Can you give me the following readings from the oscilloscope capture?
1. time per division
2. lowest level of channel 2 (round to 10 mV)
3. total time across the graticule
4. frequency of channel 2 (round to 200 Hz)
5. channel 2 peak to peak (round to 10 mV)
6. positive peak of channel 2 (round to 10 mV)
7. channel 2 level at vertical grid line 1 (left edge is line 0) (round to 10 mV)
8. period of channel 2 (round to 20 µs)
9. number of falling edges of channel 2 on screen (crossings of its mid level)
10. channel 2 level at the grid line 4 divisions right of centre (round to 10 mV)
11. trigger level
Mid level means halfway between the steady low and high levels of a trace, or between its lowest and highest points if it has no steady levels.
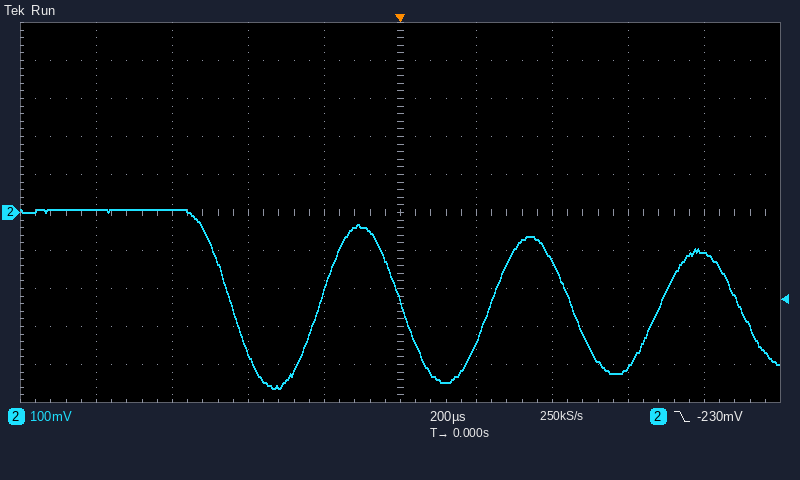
200 µs
-460 mV
2 ms
2.2 kHz
470 mV
10 mV
10 mV
440 µs
4
-110 mV
-230 mV
